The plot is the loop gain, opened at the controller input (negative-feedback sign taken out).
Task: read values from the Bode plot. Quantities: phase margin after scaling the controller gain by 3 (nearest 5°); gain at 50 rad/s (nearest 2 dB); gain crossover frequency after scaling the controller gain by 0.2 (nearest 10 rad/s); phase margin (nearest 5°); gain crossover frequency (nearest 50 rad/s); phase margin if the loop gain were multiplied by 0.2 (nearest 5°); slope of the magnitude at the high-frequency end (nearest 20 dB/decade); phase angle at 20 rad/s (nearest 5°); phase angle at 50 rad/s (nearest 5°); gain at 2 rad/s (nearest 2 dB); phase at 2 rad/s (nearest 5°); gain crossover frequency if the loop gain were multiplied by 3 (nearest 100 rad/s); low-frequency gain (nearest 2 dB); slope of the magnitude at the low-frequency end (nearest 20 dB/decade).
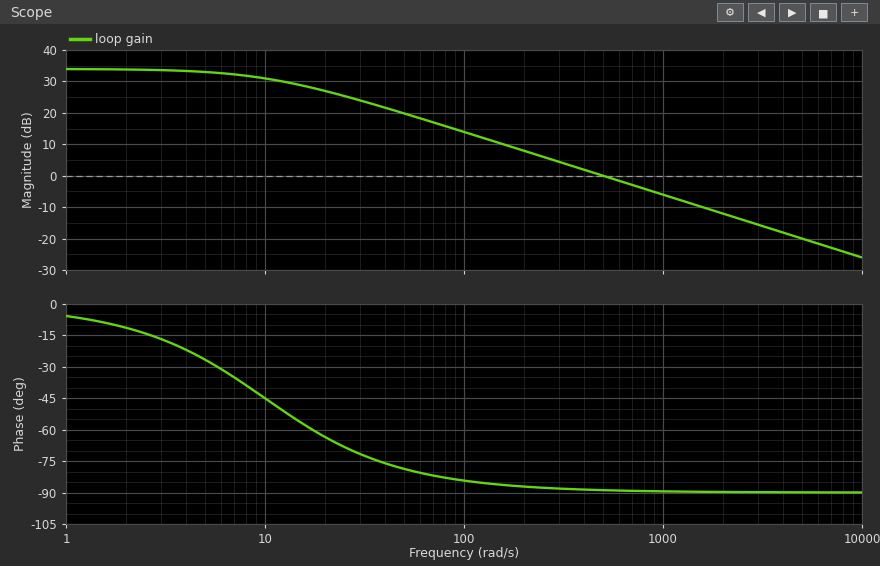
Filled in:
90°
20 dB
100 rad/s
90°
500 rad/s
95°
-20 dB/decade
-65°
-80°
34 dB
-10°
1500 rad/s
34 dB
0 dB/decade
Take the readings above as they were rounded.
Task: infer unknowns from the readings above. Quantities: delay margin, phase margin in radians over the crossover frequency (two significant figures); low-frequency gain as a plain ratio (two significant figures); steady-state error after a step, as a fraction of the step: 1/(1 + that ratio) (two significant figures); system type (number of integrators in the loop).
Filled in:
0.0031 s
50
0.020
0
